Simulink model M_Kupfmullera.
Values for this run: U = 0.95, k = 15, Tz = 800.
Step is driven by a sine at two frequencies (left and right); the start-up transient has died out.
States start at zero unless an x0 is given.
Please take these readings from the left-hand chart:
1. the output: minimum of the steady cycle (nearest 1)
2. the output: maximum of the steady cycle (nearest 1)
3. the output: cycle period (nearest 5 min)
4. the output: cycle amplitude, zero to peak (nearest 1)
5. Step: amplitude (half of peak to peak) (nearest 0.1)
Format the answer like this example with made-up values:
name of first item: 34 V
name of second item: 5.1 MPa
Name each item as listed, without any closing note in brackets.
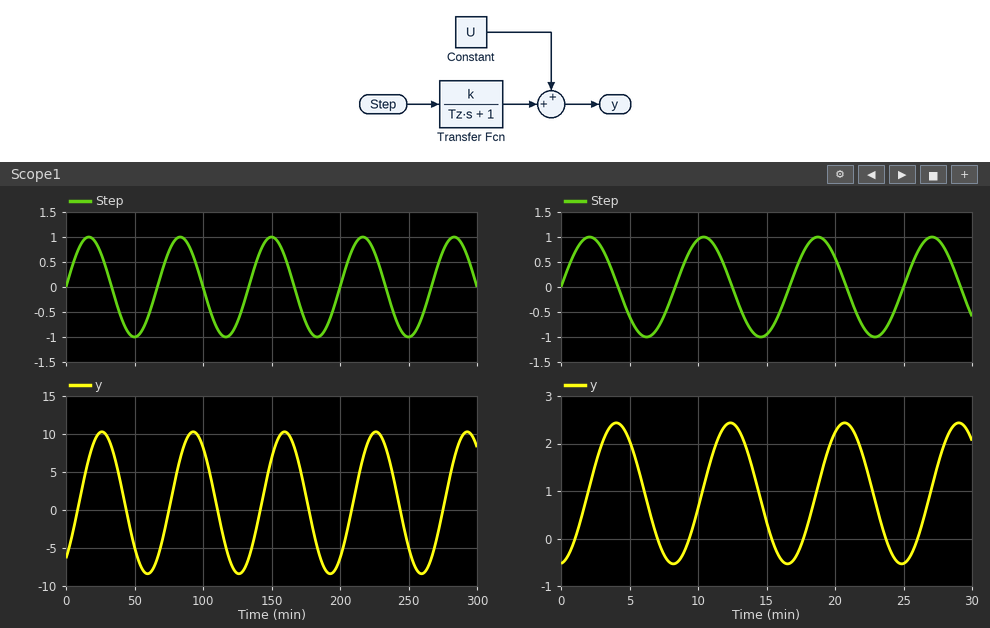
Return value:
the output: minimum of the steady cycle: -8
the output: maximum of the steady cycle: 10
the output: cycle period: 65 min
the output: cycle amplitude, zero to peak: 9
Step: amplitude (half of peak to peak): 1.0
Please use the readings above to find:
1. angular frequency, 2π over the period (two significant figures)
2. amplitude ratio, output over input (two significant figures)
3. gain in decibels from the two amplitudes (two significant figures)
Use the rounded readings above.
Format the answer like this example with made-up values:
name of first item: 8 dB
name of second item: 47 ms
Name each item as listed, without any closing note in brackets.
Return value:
angular frequency, 2π over the period: 0.097 rad/min
amplitude ratio, output over input: 9.0
gain in decibels from the two amplitudes: 19 dB
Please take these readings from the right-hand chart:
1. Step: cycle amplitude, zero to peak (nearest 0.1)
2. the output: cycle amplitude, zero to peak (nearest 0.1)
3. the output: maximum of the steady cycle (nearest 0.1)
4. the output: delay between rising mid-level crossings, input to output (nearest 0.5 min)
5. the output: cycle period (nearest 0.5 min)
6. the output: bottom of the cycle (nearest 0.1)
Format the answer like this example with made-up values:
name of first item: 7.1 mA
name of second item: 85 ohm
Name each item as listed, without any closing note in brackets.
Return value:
Step: cycle amplitude, zero to peak: 1.0
the output: cycle amplitude, zero to peak: 1.5
the output: maximum of the steady cycle: 2.4
the output: delay between rising mid-level crossings, input to output: 2.0 min
the output: cycle period: 8.5 min
the output: bottom of the cycle: -0.5
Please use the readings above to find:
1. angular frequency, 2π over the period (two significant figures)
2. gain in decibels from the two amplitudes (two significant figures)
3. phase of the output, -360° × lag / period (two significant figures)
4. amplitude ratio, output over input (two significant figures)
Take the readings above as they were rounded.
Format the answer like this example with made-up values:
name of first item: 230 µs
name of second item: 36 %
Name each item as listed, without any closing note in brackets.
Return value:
angular frequency, 2π over the period: 0.74 rad/min
gain in decibels from the two amplitudes: 3.5 dB
phase of the output, -360° × lag / period: -85°
amplitude ratio, output over input: 1.5
